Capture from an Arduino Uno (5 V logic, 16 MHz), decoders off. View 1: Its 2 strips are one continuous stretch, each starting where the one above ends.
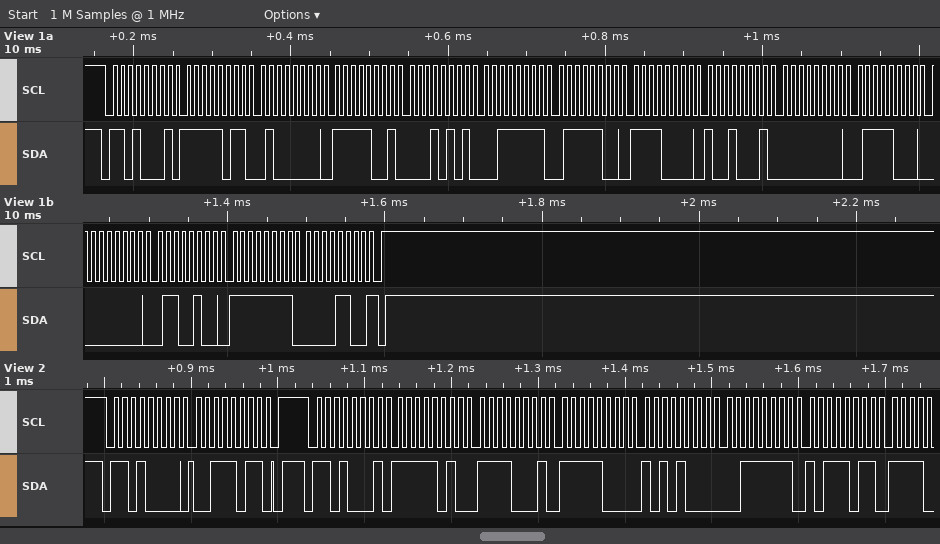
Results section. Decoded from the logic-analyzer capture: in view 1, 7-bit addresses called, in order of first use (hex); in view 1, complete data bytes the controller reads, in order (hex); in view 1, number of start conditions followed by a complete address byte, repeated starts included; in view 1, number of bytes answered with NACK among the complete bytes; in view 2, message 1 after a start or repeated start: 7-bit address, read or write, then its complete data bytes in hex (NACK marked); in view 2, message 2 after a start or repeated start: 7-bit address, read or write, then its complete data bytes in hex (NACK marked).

0x68
FB 40 F9 15 3F 7C F0 91 00 78 00 64 FF 0C
1
1
0x68 write: 3B
0x68 read: FA F1 F8 A8 3F BB
